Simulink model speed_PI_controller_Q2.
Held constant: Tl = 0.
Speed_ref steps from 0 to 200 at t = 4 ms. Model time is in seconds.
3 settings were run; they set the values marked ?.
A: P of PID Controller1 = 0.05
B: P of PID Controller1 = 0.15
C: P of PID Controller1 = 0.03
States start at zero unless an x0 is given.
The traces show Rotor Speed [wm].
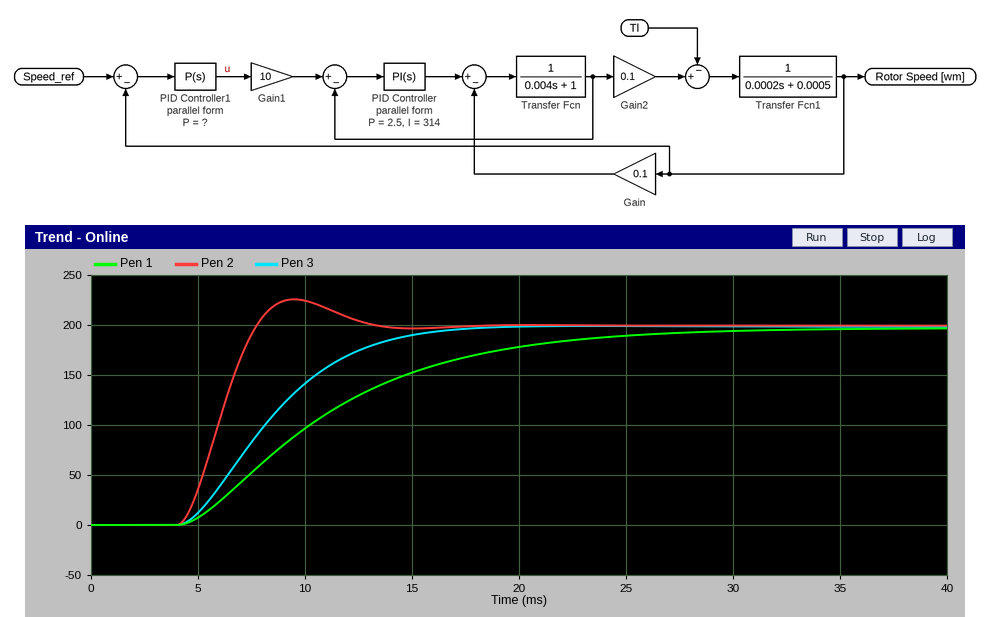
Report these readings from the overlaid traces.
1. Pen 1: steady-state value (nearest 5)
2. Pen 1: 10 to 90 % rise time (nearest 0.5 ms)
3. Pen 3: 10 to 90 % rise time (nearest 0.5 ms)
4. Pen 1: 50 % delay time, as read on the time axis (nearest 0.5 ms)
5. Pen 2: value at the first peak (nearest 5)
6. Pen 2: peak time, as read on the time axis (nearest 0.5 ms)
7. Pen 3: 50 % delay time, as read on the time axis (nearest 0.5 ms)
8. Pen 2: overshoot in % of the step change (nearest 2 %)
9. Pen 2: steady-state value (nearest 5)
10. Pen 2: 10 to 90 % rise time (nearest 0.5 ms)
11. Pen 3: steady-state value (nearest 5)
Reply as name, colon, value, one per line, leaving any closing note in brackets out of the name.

Pen 1: steady-state value: 195
Pen 1: 10 to 90 % rise time: 14.0 ms
Pen 3: 10 to 90 % rise time: 7.5 ms
Pen 1: 50 % delay time, as read on the time axis: 10.0 ms
Pen 2: value at the first peak: 225
Pen 2: peak time, as read on the time axis: 9.5 ms
Pen 3: 50 % delay time, as read on the time axis: 8.0 ms
Pen 2: overshoot in % of the step change: 14 %
Pen 2: steady-state value: 200
Pen 2: 10 to 90 % rise time: 2.5 ms
Pen 3: steady-state value: 200
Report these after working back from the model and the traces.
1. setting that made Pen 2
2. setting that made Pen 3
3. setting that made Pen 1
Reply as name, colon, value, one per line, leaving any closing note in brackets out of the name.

setting that made Pen 2: B
setting that made Pen 3: A
setting that made Pen 1: C
